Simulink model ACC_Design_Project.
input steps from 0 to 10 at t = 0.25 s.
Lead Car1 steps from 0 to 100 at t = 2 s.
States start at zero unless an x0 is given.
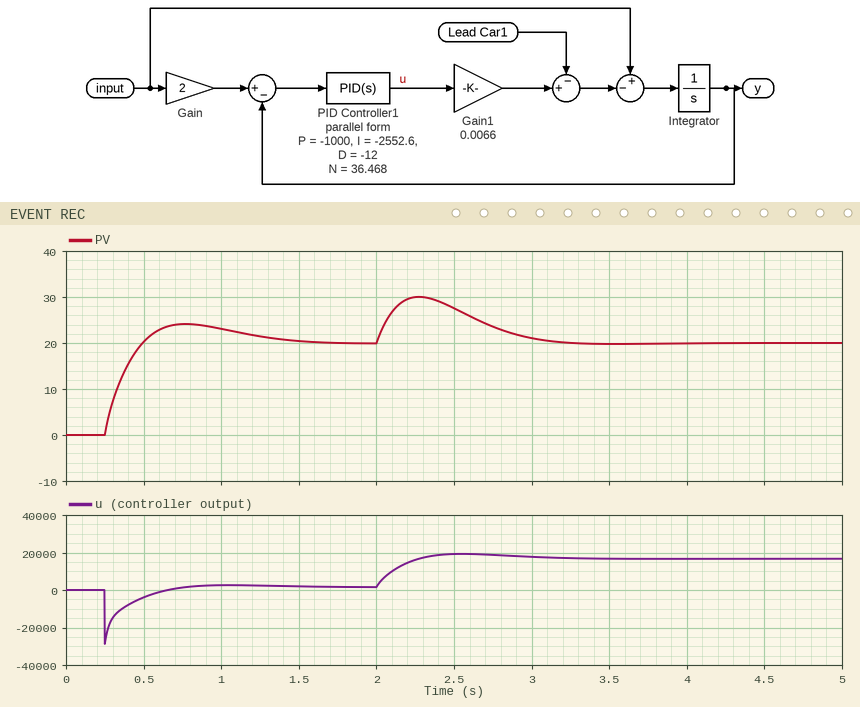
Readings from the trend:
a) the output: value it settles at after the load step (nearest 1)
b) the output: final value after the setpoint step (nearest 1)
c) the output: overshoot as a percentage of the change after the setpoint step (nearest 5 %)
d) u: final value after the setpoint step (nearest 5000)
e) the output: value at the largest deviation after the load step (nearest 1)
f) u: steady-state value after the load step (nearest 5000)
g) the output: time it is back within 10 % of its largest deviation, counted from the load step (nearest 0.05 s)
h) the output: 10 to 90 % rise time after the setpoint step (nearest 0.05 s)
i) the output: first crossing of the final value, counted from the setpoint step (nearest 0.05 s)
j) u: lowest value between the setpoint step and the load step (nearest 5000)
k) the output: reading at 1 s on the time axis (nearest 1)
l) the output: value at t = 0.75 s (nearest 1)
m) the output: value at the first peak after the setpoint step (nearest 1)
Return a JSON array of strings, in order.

["20", "20", "20 %", "0", "30", "15000", "1.00 s", "0.20 s", "0.25 s", "-30000", "23", "24", "24"]
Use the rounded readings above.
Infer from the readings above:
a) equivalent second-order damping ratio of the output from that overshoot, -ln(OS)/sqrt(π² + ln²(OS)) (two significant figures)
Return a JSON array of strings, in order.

["0.46"]
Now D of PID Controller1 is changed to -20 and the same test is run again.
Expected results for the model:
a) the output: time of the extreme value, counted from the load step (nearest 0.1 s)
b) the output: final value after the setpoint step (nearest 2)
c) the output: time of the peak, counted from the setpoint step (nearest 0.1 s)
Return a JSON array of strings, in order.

["0.3 s", "20", "0.5 s"]
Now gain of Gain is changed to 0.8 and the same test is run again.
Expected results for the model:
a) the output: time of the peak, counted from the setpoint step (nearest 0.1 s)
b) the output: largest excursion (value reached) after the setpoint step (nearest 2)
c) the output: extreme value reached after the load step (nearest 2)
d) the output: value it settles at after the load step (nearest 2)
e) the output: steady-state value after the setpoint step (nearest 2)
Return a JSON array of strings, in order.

["0.5 s", "10", "18", "8", "8"]
